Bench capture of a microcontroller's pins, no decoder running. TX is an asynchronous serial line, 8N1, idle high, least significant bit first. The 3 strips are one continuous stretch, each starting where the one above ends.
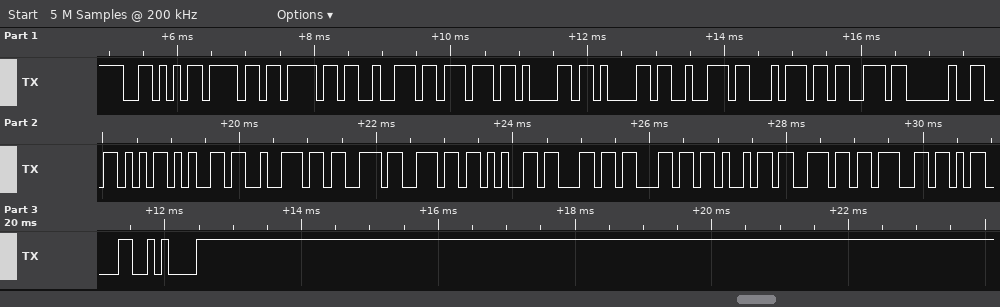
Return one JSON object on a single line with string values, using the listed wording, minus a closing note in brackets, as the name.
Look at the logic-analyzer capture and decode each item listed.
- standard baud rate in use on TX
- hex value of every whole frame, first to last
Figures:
{"standard baud rate in use on TX": "9600 baud", "hex value of every whole frame, first to last": "56 6F 6F 72 77 61 61 72 74 73 20 56 65 72 73 6E 65 6C 6C 69 6E 67 0D 0A"}
